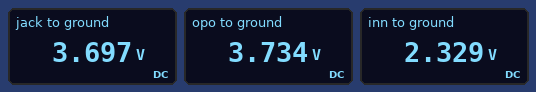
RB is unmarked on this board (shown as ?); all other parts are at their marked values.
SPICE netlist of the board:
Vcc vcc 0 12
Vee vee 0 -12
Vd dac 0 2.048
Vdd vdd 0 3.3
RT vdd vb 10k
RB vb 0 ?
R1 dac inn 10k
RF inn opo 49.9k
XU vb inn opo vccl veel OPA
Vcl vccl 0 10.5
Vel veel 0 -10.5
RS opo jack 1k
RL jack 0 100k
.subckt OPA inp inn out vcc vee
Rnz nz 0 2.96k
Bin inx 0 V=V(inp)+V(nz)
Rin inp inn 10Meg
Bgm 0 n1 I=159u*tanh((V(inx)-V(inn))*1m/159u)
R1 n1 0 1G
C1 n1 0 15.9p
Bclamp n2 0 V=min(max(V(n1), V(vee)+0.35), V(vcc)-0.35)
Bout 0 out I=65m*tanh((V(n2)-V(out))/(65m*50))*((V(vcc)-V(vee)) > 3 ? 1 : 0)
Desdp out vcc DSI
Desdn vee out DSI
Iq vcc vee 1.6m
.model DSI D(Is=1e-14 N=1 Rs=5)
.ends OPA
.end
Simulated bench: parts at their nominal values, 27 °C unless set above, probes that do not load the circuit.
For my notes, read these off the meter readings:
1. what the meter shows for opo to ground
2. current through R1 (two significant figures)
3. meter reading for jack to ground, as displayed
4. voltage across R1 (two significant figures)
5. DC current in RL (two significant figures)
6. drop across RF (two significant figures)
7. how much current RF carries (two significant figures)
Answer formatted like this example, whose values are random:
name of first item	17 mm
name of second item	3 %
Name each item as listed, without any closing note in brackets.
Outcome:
what the meter shows for opo to ground	3.734 V
current through R1	28 µA
meter reading for jack to ground, as displayed	3.697 V
voltage across R1	280 mV
DC current in RL	37 µA
drop across RF	1.4 V
how much current RF carries	28 µA
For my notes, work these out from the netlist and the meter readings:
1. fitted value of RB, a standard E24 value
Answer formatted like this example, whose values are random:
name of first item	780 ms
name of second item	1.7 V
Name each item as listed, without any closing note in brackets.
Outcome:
fitted value of RB, a standard E24 value	24 kΩ
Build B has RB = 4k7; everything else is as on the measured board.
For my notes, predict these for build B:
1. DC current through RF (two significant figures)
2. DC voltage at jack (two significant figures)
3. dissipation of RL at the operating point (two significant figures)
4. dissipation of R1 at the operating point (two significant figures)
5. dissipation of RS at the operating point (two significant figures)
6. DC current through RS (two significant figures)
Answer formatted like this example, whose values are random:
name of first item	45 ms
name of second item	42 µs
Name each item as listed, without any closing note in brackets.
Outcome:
DC current through RF	99 µA
DC voltage at jack	-3.9 V
dissipation of RL at the operating point	150 µW
dissipation of R1 at the operating point	99 µW
dissipation of RS at the operating point	1.5 µW
DC current through RS	39 µA
